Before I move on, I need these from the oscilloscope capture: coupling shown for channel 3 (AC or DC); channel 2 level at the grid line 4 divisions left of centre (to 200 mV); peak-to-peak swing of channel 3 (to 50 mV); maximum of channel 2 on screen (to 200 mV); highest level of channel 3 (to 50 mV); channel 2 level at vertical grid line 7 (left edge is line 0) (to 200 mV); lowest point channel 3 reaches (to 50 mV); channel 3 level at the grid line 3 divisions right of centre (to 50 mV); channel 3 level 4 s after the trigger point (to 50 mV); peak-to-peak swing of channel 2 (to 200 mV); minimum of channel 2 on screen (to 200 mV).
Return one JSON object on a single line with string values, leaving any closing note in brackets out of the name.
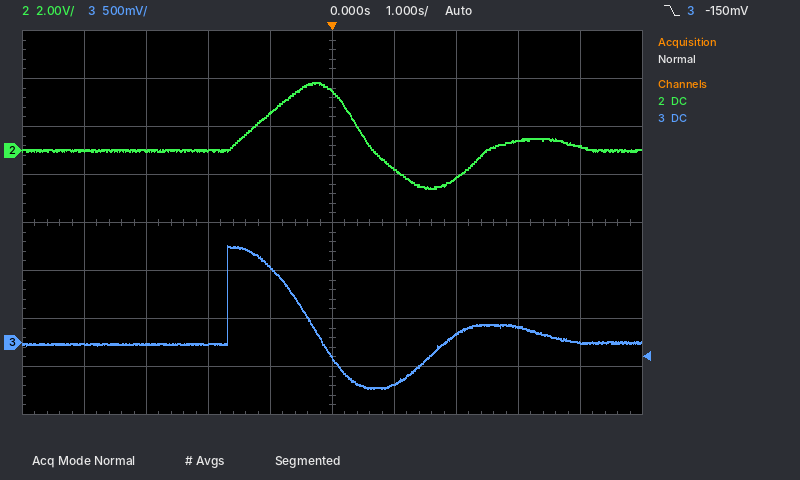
{"coupling shown for channel 3": "DC", "channel 2 level at the grid line 4 divisions left of centre": "0.0 V", "peak-to-peak swing of channel 3": "1.50 V", "maximum of channel 2 on screen": "2.8 V", "highest level of channel 3": "1.00 V", "channel 2 level at vertical grid line 7 (left edge is line 0)": "-1.2 V", "lowest point channel 3 reaches": "-500 mV", "channel 3 level at the grid line 3 divisions right of centre": "150 mV", "channel 3 level 4 s after the trigger point": "0 mV", "peak-to-peak swing of channel 2": "4.4 V", "minimum of channel 2 on screen": "-1.6 V"}
